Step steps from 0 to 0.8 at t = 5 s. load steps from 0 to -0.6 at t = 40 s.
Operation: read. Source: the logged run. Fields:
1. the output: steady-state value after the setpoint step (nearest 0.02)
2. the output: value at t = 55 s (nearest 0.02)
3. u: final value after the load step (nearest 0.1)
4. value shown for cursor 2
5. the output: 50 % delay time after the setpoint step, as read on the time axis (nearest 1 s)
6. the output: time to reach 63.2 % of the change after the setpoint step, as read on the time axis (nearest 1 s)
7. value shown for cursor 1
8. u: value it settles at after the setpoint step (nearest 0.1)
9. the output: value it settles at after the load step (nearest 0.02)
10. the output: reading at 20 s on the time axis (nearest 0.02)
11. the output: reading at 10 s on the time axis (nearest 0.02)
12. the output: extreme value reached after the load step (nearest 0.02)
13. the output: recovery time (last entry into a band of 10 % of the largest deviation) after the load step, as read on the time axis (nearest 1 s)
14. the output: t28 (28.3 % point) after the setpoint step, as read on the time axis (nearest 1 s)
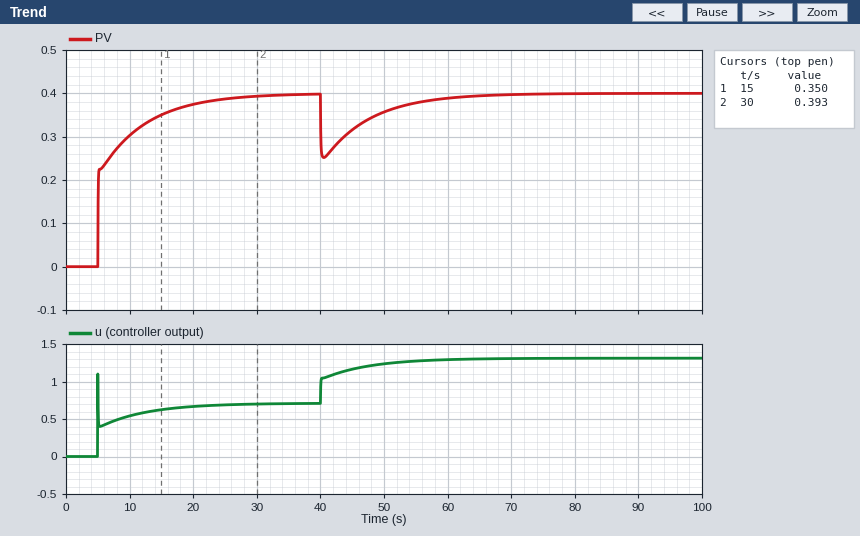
0.40
0.38
1.3
0.393
5 s
7 s
0.350
0.7
0.40
0.38
0.30
0.26
58 s
5 s
